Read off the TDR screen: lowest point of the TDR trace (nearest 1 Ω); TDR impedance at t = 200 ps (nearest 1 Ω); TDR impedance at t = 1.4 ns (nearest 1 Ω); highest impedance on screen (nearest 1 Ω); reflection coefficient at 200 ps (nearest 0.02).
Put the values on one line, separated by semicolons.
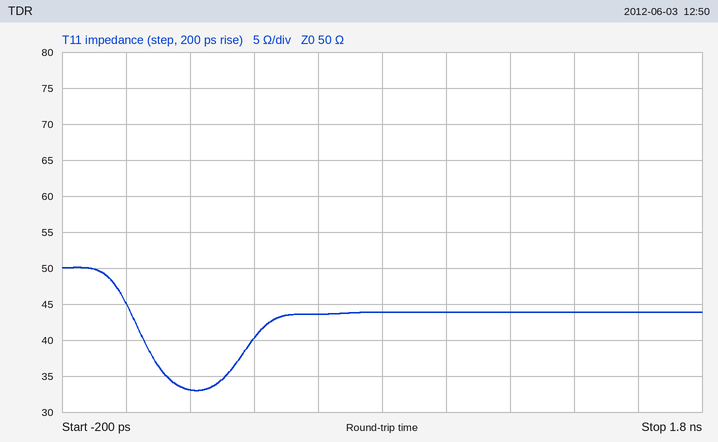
33 Ω; 33 Ω; 44 Ω; 50 Ω; -0.20
